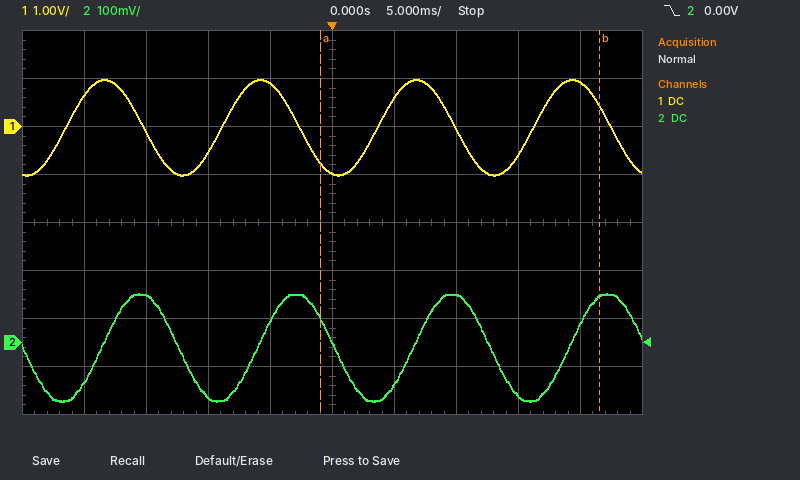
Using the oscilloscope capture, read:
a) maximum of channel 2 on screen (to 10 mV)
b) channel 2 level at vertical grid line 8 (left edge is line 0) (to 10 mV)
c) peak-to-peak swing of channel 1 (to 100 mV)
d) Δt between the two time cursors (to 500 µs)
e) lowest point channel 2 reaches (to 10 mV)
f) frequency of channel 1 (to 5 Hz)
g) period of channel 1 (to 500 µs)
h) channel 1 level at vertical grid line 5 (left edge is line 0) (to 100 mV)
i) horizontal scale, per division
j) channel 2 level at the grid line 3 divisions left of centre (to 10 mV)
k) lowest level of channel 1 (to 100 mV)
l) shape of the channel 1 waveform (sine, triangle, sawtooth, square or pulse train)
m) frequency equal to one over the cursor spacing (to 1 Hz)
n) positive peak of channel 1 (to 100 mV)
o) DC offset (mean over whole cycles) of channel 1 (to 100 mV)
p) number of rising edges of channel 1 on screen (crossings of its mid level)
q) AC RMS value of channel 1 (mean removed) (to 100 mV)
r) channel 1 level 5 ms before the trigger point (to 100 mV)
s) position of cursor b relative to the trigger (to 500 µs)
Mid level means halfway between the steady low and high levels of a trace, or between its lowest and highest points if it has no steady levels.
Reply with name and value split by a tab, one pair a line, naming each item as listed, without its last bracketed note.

maximum of channel 2 on screen	100 mV
channel 2 level at vertical grid line 8 (left edge is line 0)	-110 mV
peak-to-peak swing of channel 1	2.0 V
Δt between the two time cursors	22.5 ms
lowest point channel 2 reaches	-120 mV
frequency of channel 1	80 Hz
period of channel 1	12.5 ms
channel 1 level at vertical grid line 5 (left edge is line 0)	-1.0 V
horizontal scale, per division	5 ms
channel 2 level at the grid line 3 divisions left of centre	100 mV
lowest level of channel 1	-1.0 V
shape of the channel 1 waveform	sine
frequency equal to one over the cursor spacing	44 Hz
positive peak of channel 1	1.0 V
DC offset (mean over whole cycles) of channel 1	0.0 V
number of rising edges of channel 1 on screen	4
AC RMS value of channel 1 (mean removed)	700 mV
channel 1 level 5 ms before the trigger point	900 mV
position of cursor b relative to the trigger	+21.5 ms
